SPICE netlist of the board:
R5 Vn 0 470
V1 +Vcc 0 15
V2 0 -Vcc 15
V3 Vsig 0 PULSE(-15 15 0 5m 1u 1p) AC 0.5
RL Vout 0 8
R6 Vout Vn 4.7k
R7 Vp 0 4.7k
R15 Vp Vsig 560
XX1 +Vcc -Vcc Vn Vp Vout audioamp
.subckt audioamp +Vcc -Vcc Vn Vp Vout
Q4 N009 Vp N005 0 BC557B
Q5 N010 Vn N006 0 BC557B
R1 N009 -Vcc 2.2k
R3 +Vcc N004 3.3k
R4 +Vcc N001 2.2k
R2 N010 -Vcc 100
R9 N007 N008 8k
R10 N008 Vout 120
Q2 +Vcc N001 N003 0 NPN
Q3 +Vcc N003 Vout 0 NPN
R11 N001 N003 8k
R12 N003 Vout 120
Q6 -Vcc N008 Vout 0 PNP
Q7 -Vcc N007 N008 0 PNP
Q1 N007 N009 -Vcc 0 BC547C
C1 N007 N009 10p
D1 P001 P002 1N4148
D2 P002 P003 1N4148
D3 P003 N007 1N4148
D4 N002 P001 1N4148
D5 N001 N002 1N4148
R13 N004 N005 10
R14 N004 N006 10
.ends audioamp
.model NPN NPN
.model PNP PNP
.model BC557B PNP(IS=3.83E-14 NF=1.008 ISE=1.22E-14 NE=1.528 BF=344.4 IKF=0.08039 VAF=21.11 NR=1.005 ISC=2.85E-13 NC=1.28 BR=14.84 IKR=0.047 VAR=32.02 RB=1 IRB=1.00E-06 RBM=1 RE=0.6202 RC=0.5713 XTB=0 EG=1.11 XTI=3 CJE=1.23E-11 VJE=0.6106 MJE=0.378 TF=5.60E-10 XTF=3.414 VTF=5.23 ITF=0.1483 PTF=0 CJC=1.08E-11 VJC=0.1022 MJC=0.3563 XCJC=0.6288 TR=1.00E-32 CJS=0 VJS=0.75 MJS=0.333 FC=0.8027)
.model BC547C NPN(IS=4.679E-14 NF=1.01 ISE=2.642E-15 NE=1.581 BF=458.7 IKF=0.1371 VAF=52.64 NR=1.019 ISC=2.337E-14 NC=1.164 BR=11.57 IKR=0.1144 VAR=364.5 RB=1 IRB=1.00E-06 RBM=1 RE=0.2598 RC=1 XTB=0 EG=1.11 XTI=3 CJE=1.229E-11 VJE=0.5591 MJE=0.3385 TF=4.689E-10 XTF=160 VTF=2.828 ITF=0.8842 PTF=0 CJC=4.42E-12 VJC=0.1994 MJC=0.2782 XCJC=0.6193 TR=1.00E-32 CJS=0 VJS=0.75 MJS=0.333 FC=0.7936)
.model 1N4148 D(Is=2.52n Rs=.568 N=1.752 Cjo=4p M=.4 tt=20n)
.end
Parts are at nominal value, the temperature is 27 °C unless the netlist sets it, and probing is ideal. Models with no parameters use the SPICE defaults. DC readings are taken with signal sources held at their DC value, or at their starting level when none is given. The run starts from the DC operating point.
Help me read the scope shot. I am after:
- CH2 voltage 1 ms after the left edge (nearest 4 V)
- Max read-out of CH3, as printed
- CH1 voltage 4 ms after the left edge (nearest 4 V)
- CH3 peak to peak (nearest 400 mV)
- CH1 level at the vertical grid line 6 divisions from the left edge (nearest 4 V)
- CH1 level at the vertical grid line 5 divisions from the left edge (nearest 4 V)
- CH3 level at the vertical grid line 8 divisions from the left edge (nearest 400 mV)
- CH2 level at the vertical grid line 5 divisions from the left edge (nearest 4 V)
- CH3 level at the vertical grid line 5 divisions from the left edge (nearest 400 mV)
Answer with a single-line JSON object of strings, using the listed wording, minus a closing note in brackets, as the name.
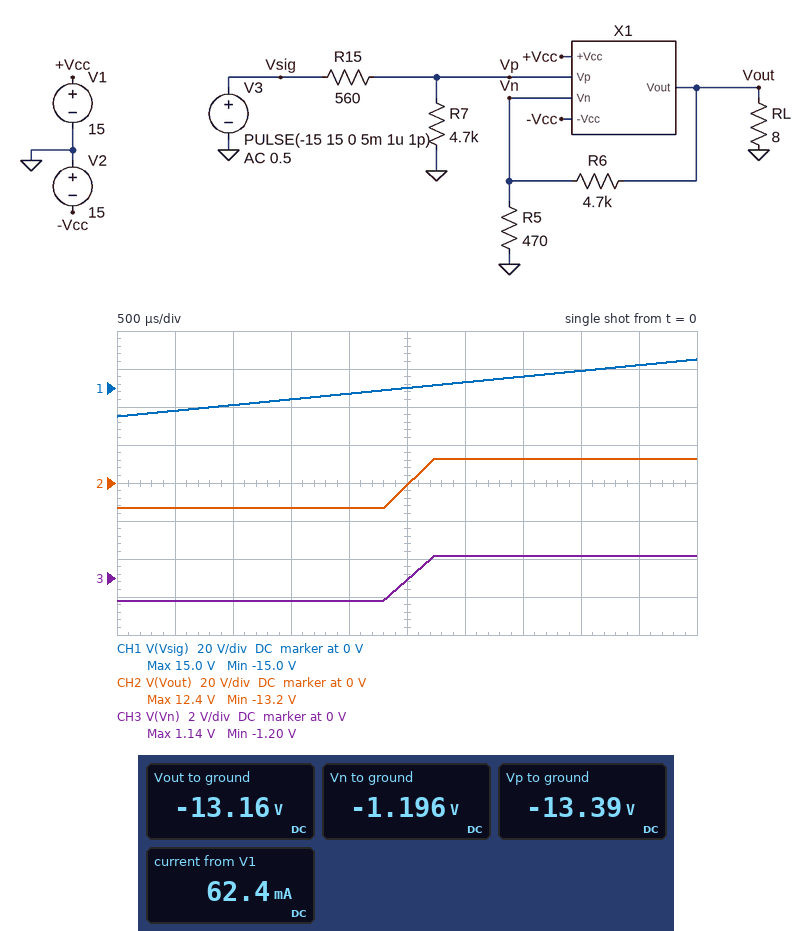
{"CH2 voltage 1 ms after the left edge": "-12 V", "Max read-out of CH3, as printed": "1.14 V", "CH1 voltage 4 ms after the left edge": "8 V", "CH3 peak to peak": "2.4 V", "CH1 level at the vertical grid line 6 divisions from the left edge": "4 V", "CH1 level at the vertical grid line 5 divisions from the left edge": "0 V", "CH3 level at the vertical grid line 8 divisions from the left edge": "1.2 V", "CH2 level at the vertical grid line 5 divisions from the left edge": "0 V", "CH3 level at the vertical grid line 5 divisions from the left edge": "0 V"}
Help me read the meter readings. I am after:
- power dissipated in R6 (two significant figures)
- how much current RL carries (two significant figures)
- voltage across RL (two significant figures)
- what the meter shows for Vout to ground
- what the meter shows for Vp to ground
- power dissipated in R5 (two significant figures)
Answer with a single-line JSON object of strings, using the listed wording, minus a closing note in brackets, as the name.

{"power dissipated in R6": "30 mW", "how much current RL carries": "1.6 A", "voltage across RL": "13 V", "what the meter shows for Vout to ground": "-13.16 V", "what the meter shows for Vp to ground": "-13.39 V", "power dissipated in R5": "3.0 mW"}
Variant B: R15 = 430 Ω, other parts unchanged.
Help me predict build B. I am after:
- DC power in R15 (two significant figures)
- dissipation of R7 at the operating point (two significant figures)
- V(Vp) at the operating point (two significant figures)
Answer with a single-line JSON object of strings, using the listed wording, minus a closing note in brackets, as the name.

{"DC power in R15": "3.7 mW", "dissipation of R7 at the operating point": "40 mW", "V(Vp) at the operating point": "-14 V"}
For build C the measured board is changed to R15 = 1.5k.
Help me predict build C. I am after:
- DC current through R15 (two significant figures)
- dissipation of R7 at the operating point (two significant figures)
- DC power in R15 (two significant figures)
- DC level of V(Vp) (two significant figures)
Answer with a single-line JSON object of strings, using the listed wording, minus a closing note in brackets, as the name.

{"DC current through R15": "2.4 mA", "dissipation of R7 at the operating point": "27 mW", "DC power in R15": "8.9 mW", "DC level of V(Vp)": "-11 V"}
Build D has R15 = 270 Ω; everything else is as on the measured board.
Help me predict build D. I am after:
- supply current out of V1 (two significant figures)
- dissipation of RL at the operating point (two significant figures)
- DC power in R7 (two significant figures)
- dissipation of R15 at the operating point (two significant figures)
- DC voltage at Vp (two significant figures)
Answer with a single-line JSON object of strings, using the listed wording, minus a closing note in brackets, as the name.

{"supply current out of V1": "63 mA", "dissipation of RL at the operating point": "22 W", "DC power in R7": "43 mW", "dissipation of R15 at the operating point": "2.5 mW", "DC voltage at Vp": "-14 V"}
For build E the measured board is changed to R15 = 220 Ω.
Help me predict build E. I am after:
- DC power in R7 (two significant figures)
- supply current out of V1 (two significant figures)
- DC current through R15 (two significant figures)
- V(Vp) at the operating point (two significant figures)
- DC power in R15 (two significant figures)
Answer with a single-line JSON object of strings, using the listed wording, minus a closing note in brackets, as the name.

{"DC power in R7": "44 mW", "supply current out of V1": "63 mA", "DC current through R15": "3.1 mA", "V(Vp) at the operating point": "-14 V", "DC power in R15": "2.1 mW"}
